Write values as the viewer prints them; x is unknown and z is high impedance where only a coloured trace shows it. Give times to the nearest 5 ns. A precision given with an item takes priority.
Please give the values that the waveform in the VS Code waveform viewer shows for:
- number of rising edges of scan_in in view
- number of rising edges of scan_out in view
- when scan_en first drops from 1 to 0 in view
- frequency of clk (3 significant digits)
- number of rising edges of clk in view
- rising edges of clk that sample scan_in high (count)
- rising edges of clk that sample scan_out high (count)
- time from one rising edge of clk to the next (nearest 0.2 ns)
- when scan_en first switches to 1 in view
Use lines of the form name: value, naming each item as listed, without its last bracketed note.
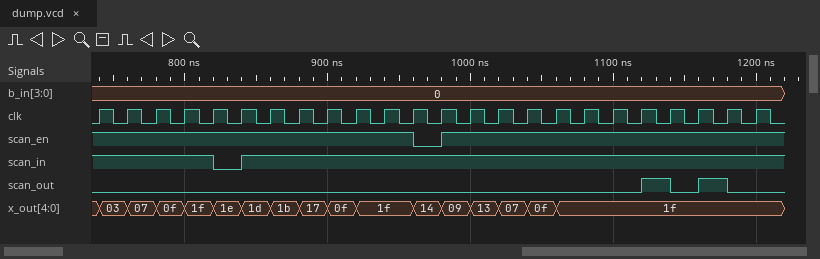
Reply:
number of rising edges of scan_in in view: 1
number of rising edges of scan_out in view: 2
when scan_en first drops from 1 to 0 in view: 960 ns
frequency of clk: 50.0 MHz
number of rising edges of clk in view: 24
rising edges of clk that sample scan_in high: 23
rising edges of clk that sample scan_out high: 2
time from one rising edge of clk to the next: 20 ns
when scan_en first switches to 1 in view: 980 ns
